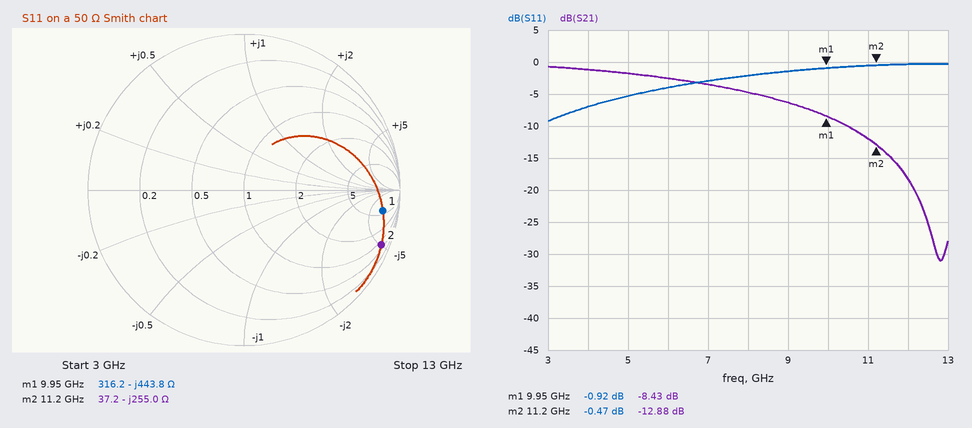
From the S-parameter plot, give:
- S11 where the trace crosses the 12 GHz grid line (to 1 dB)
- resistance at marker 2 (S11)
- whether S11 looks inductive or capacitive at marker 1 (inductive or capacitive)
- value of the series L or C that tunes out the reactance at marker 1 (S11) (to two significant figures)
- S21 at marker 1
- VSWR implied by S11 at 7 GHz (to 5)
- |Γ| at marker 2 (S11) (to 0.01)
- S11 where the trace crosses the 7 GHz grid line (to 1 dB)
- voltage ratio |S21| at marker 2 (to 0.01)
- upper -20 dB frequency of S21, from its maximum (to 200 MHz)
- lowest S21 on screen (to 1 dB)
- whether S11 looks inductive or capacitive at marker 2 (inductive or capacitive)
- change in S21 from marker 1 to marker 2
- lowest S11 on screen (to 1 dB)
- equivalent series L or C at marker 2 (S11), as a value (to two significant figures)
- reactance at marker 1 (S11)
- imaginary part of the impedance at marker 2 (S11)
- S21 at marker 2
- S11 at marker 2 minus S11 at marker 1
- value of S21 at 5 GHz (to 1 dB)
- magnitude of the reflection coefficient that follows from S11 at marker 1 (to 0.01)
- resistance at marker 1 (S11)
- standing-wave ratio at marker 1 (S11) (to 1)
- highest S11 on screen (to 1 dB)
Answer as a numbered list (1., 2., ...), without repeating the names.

1. 0 dB
2. 37.2 Ω
3. capacitive
4. 7.1 nH
5. -8.43 dB
6. 5
7. 0.95
8. -3 dB
9. 0.23
10. 12.2 GHz
11. -31 dB
12. capacitive
13. -4.45 dB
14. -9 dB
15. 56 fF
16. -443.8 Ω
17. -255.0 Ω
18. -12.88 dB
19. 0.45 dB
20. -2 dB
21. 0.90
22. 316.2 Ω
23. 19
24. 0 dB
